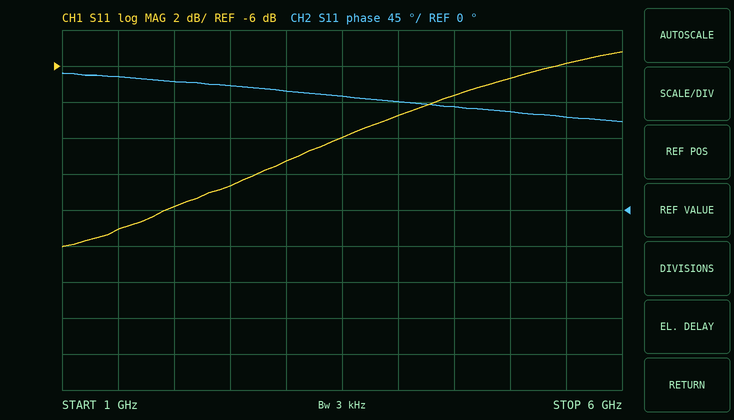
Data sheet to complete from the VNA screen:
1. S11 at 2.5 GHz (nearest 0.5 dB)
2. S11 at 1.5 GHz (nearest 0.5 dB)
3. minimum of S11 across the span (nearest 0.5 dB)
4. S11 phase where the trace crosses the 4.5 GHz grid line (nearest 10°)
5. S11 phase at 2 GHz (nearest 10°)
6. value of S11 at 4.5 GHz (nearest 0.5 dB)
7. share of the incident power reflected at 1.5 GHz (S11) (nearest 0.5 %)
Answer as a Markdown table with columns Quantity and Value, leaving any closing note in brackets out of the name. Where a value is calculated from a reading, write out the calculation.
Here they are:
| Quantity | Value |
|---|---|
| S11 at 2.5 GHz | -12.5 dB |
| S11 at 1.5 GHz | -15.0 dB |
| minimum of S11 across the span | -16.0 dB |
| S11 phase where the trace crosses the 4.5 GHz grid line | 130° |
| S11 phase at 2 GHz | 160° |
| value of S11 at 4.5 GHz | -7.5 dB |
| share of the incident power reflected at 1.5 GHz (S11) | 10^(-15/10) ≈ 3.16 %, so 3.0 % to the nearest 0.5 % |
